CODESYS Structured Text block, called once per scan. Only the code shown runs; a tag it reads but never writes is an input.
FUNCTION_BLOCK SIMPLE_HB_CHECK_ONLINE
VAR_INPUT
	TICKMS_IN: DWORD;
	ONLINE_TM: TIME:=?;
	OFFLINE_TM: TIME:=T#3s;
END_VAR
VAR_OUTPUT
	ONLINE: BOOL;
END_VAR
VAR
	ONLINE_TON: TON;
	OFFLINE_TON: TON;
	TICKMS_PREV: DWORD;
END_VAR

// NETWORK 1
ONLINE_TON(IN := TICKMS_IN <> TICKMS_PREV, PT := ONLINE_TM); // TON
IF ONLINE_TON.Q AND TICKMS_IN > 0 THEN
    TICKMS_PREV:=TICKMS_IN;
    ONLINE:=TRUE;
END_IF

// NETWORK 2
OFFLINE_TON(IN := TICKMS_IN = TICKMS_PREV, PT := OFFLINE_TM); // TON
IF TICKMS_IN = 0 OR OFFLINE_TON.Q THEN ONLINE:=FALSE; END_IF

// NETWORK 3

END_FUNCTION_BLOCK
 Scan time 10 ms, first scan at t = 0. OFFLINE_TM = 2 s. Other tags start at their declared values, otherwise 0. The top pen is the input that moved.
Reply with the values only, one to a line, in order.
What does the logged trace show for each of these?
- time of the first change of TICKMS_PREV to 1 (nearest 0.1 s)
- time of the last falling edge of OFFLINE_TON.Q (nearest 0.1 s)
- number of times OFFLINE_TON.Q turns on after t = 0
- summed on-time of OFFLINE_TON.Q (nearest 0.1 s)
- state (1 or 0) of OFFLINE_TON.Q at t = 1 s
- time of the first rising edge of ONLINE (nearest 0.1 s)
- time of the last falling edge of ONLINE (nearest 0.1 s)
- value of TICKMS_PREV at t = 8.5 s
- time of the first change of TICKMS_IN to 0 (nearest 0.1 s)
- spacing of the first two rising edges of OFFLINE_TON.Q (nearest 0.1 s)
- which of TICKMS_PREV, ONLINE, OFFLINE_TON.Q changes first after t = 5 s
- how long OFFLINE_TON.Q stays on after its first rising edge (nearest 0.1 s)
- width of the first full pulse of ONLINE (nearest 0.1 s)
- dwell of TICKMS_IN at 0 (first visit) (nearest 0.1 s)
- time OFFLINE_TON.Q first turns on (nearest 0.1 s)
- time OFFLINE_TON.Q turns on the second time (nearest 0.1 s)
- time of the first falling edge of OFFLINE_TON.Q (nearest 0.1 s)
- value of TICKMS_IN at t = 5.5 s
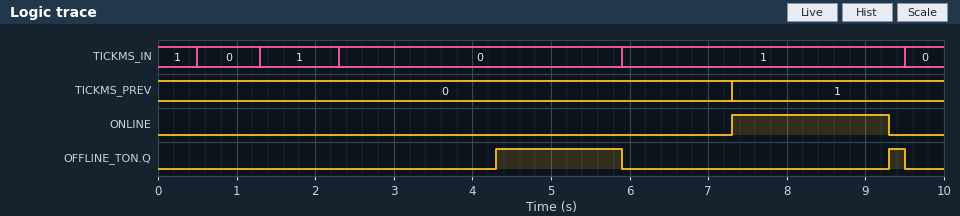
7.3 s
9.5 s
2
1.8 s
0
7.3 s
9.3 s
1
0.5 s
5.0 s
OFFLINE_TON.Q
1.6 s
2.0 s
0.8 s
4.3 s
9.3 s
5.9 s
0
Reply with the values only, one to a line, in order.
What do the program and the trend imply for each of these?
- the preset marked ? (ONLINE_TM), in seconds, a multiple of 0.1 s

1.4 s
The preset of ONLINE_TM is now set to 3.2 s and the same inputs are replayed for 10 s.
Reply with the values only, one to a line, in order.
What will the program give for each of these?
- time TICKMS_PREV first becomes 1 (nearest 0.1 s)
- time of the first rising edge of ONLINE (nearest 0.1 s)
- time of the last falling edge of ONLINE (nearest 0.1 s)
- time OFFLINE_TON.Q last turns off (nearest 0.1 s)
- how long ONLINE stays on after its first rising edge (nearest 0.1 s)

9.1 s
9.1 s
9.5 s
5.9 s
0.4 s
